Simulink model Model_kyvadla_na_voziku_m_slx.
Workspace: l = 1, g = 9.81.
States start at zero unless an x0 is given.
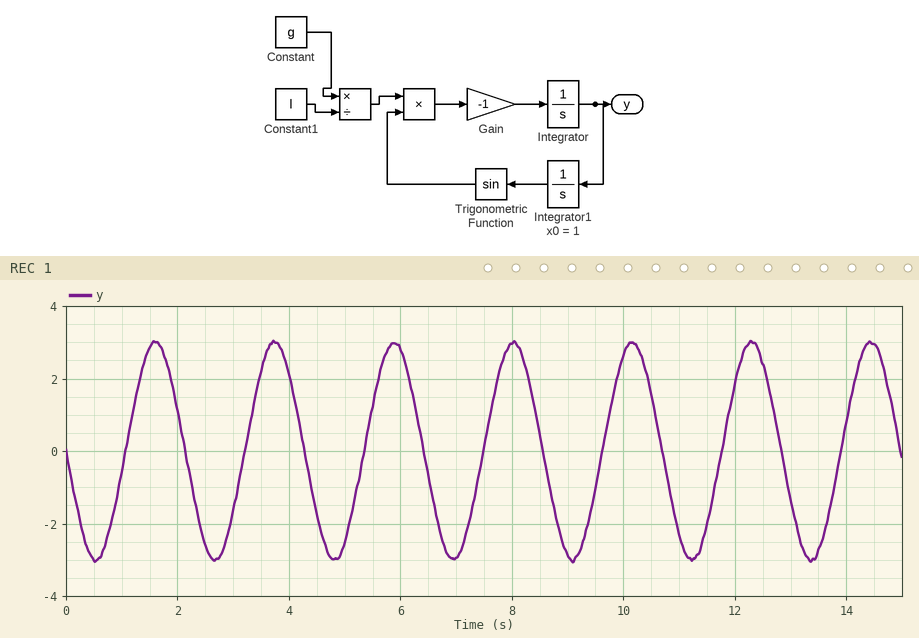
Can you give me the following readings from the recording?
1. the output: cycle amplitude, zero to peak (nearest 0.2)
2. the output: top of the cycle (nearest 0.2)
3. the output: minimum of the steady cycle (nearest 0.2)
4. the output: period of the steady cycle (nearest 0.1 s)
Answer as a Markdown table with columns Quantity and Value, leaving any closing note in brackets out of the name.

| Quantity | Value |
|---|---|
| the output: cycle amplitude, zero to peak | 3.0 |
| the output: top of the cycle | 3.0 |
| the output: minimum of the steady cycle | -3.0 |
| the output: period of the steady cycle | 2.1 s |
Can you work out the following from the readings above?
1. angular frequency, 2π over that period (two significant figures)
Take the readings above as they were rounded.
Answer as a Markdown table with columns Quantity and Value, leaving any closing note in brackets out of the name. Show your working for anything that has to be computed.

| Quantity | Value |
|---|---|
| angular frequency, 2π over that period | 2π / 2.1 = 3.0 rad/s |
